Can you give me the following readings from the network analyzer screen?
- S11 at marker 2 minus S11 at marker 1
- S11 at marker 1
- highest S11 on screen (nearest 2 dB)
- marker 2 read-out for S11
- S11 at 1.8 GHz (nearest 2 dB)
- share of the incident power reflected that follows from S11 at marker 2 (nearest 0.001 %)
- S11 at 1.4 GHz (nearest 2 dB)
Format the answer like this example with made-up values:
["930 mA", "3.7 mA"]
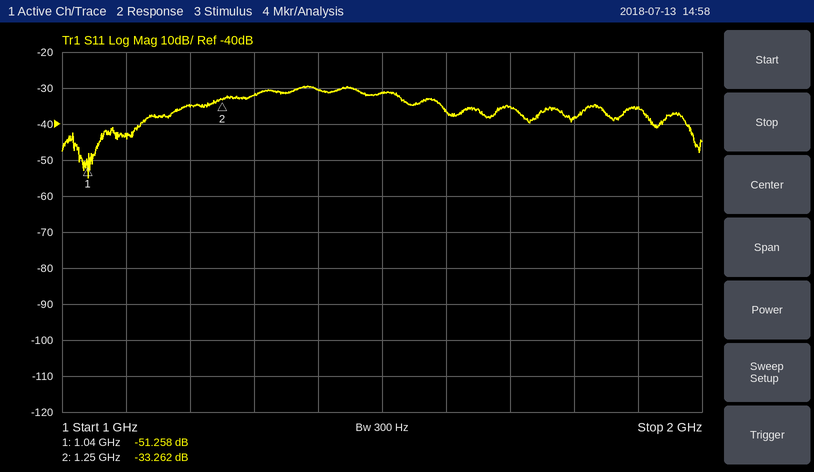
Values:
["17.996 dB", "-51.258 dB", "-30 dB", "-33.262 dB", "-38 dB", "0.047 %", "-30 dB"]
